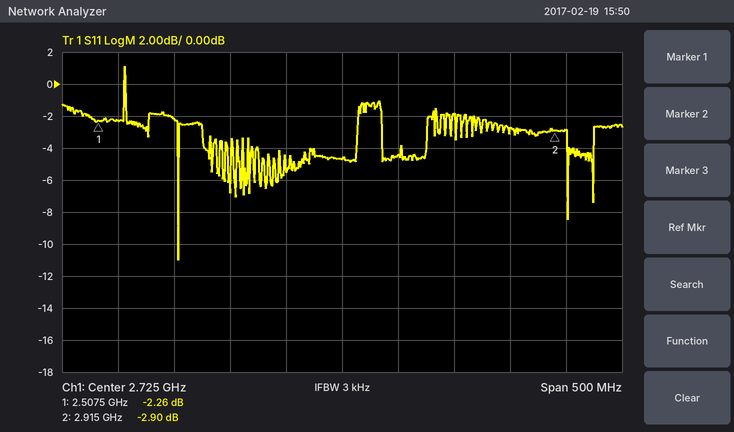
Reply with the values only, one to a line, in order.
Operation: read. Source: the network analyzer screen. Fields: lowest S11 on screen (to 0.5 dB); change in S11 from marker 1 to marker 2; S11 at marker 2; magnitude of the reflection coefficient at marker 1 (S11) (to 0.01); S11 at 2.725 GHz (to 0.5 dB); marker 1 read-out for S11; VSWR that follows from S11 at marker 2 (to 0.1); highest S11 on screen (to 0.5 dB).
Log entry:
-11.0 dB
-0.64 dB
-2.90 dB
0.77
-4.5 dB
-2.26 dB
6.0
1.0 dB
